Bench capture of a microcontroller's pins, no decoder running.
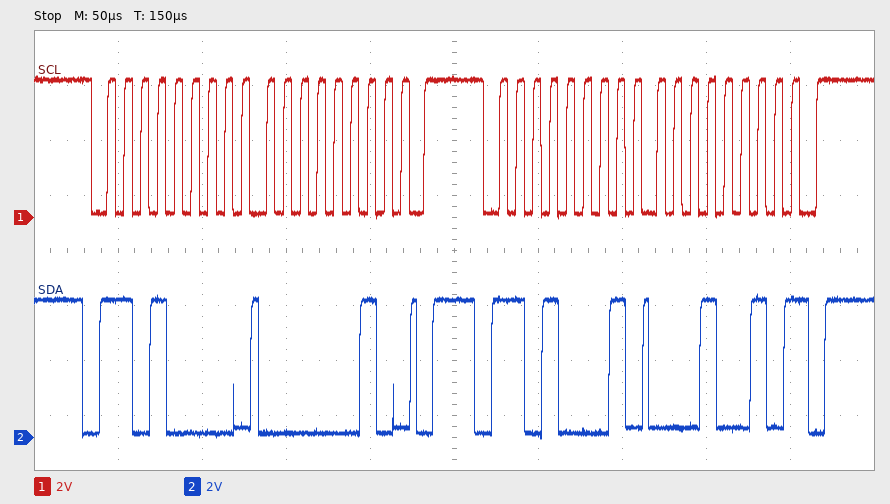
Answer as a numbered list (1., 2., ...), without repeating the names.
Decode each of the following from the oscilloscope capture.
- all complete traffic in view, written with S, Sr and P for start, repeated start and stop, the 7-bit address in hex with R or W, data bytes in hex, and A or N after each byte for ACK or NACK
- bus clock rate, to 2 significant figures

1. S 68W A 02 A P S 68R A 12 N P
2. 100 kHz
